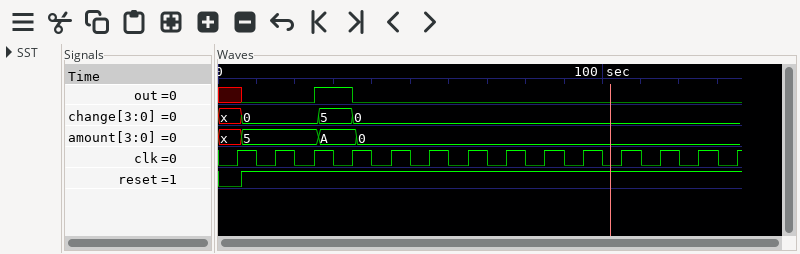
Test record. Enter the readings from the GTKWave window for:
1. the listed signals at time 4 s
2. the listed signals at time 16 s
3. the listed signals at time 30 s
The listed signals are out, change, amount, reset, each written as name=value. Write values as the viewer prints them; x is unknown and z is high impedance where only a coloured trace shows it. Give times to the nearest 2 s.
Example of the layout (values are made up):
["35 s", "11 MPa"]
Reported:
["out=x, change=x, amount=x, reset=0", "out=0, change=0, amount=5, reset=1", "out=1, change=5, amount=A, reset=1"]
